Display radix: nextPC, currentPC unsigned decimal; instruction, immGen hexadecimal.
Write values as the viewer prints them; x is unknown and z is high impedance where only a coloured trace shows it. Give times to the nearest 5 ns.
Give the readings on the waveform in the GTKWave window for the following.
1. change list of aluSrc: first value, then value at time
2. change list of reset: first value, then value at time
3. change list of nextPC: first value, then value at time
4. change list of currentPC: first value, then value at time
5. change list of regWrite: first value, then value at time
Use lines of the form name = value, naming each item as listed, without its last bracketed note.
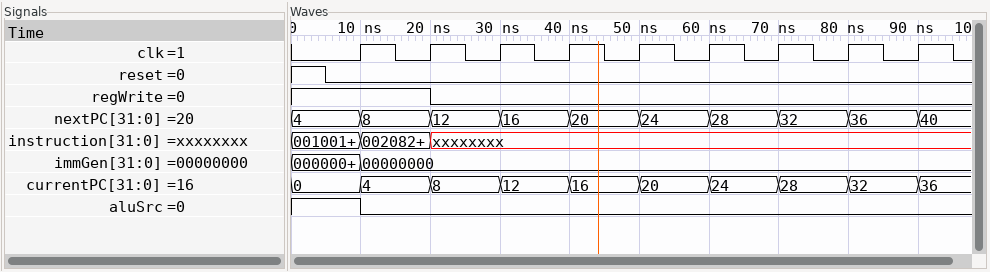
change list of aluSrc: first value, then value at time = 1, 0 at 10 ns
change list of reset: first value, then value at time = 1, 0 at 5 ns
change list of nextPC: first value, then value at time = 4, 8 at 10 ns, 12 at 20 ns, 16 at 30 ns, 20 at 40 ns, 24 at 50 ns, 28 at 60 ns, 32 at 70 ns, 36 at 80 ns, 40 at 90 ns
change list of currentPC: first value, then value at time = 0, 4 at 10 ns, 8 at 20 ns, 12 at 30 ns, 16 at 40 ns, 20 at 50 ns, 24 at 60 ns, 28 at 70 ns, 32 at 80 ns, 36 at 90 ns
change list of regWrite: first value, then value at time = 1, 0 at 20 ns
